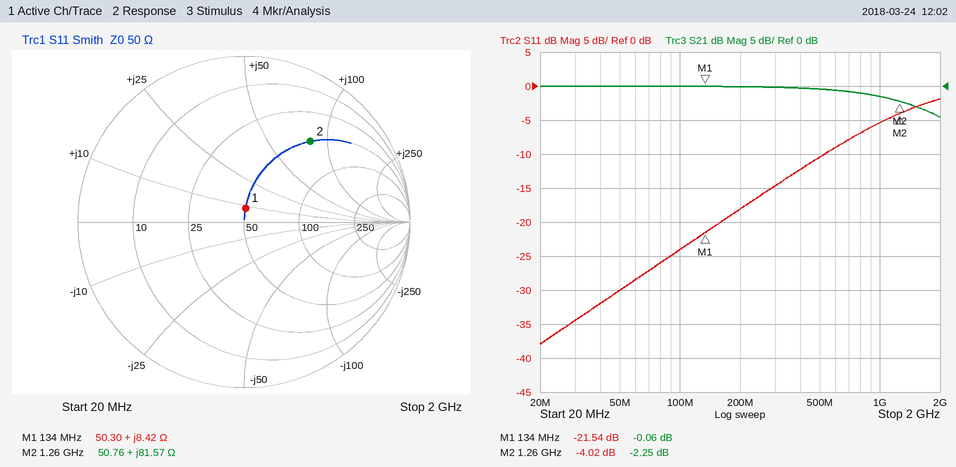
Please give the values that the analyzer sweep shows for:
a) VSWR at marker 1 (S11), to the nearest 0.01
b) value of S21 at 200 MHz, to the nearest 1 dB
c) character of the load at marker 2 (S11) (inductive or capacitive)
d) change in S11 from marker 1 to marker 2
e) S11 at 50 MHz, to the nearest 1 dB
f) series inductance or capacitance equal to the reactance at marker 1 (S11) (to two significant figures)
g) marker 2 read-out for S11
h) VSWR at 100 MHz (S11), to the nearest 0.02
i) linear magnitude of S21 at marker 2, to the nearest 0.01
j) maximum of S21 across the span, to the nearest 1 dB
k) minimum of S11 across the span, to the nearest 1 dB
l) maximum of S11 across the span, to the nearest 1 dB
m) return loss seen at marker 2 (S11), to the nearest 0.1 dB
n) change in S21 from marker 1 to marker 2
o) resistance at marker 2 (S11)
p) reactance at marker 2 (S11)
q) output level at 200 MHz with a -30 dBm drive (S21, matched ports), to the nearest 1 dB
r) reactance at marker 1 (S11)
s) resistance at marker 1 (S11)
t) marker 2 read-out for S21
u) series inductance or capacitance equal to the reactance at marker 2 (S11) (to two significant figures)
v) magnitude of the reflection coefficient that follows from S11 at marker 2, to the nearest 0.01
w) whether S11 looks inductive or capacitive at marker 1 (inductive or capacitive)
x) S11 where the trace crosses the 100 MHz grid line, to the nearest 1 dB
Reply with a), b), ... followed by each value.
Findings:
a) 1.18
b) 0 dB
c) inductive
d) 17.52 dB
e) -30 dB
f) 10 nH
g) -4.02 dB
h) 1.14
i) 0.77
j) 0 dB
k) -38 dB
l) -2 dB
m) 4.0 dB
n) -2.19 dB
o) 50.76 Ω
p) +81.57 Ω
q) -30 dBm
r) +8.42 Ω
s) 50.30 Ω
t) -2.25 dB
u) 10 nH
v) 0.63
w) inductive
x) -24 dB
